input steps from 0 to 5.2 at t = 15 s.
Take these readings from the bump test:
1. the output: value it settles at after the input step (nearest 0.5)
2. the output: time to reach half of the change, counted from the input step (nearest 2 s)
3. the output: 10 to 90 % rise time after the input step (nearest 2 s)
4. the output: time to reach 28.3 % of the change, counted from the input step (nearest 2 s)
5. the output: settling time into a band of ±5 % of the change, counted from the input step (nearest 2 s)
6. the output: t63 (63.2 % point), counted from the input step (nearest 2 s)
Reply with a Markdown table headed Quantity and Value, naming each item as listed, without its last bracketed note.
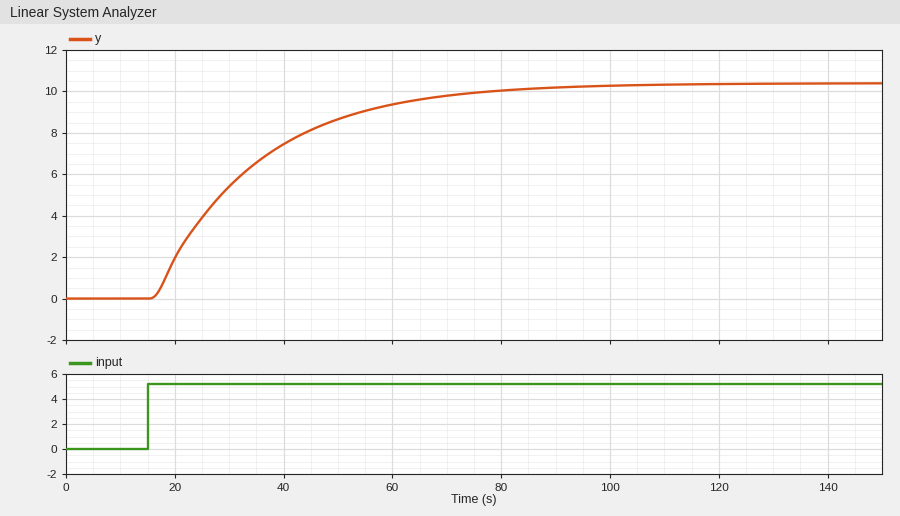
| Quantity | Value |
|---|---|
| the output: value it settles at after the input step | 10.5 |
| the output: time to reach half of the change, counted from the input step | 14 s |
| the output: 10 to 90 % rise time after the input step | 42 s |
| the output: time to reach 28.3 % of the change, counted from the input step | 8 s |
| the output: settling time into a band of ±5 % of the change, counted from the input step | 58 s |
| the output: t63 (63.2 % point), counted from the input step | 20 s |
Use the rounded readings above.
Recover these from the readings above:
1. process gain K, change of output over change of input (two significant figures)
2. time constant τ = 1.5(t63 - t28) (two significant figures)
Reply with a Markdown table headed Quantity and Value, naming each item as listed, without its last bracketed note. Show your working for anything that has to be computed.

| Quantity | Value |
|---|---|
| process gain K, change of output over change of input | (10.5 - 0) / 5.2 = 2.0 |
| time constant τ = 1.5(t63 - t28) | 1.5 × (20 - 8) = 18 s |
